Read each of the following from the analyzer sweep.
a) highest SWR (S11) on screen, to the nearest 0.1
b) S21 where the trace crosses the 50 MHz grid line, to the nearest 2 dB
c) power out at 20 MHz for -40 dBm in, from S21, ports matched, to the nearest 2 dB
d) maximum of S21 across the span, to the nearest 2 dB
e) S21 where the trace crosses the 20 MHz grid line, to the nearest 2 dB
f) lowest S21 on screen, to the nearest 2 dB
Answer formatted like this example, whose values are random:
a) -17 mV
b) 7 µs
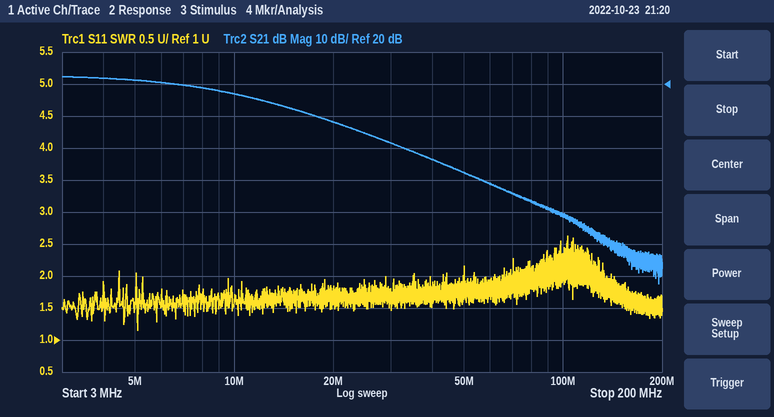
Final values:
a) 2.6
b) -8 dB
c) -32 dBm
d) 22 dB
e) 8 dB
f) -42 dB
